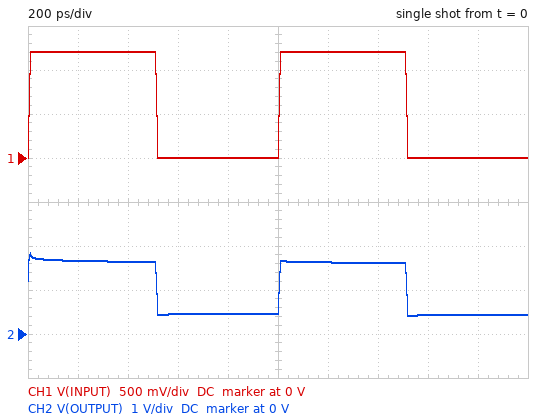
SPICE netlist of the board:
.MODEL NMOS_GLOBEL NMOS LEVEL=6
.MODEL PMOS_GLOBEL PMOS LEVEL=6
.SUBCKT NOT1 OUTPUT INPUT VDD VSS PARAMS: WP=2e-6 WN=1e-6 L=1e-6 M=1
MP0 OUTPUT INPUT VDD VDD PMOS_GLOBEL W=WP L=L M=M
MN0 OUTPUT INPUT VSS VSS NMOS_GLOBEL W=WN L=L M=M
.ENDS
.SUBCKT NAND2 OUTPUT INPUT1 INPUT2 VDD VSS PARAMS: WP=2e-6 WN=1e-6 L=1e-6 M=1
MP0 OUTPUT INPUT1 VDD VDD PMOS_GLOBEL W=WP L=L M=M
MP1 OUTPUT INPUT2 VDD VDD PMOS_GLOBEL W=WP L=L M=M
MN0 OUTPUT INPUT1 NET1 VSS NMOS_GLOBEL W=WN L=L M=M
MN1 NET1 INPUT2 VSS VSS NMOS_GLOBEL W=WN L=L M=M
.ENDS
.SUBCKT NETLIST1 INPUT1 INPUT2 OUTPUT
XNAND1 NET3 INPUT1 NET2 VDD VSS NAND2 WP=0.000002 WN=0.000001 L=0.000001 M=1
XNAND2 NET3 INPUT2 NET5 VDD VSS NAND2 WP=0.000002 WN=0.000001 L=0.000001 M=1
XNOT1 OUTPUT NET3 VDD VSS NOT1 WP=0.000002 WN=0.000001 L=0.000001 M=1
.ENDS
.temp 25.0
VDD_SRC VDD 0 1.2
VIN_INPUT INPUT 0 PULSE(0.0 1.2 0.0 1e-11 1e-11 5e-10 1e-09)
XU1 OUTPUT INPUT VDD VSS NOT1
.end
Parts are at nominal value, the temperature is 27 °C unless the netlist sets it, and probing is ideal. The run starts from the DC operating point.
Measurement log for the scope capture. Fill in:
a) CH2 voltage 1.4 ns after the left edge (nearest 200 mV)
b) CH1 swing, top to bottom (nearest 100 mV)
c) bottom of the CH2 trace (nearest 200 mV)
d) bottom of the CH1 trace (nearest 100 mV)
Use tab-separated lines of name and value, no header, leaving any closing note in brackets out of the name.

CH2 voltage 1.4 ns after the left edge	1.6 V
CH1 swing, top to bottom	1.2 V
bottom of the CH2 trace	400 mV
bottom of the CH1 trace	0 V
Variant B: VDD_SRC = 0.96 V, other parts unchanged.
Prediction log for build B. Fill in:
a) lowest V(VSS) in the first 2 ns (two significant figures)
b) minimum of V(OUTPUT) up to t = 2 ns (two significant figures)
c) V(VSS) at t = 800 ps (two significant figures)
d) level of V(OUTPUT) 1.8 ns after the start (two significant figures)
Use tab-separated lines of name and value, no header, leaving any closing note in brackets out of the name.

lowest V(VSS) in the first 2 ns	560 mV
minimum of V(OUTPUT) up to t = 2 ns	180 mV
V(VSS) at t = 800 ps	590 mV
level of V(OUTPUT) 1.8 ns after the start	190 mV
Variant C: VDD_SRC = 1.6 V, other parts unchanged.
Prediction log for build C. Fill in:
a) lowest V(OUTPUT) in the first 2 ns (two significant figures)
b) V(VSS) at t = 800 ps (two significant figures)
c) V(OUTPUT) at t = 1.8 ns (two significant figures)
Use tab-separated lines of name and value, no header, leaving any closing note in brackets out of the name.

lowest V(OUTPUT) in the first 2 ns	820 mV
V(VSS) at t = 800 ps	1.2 V
V(OUTPUT) at t = 1.8 ns	830 mV
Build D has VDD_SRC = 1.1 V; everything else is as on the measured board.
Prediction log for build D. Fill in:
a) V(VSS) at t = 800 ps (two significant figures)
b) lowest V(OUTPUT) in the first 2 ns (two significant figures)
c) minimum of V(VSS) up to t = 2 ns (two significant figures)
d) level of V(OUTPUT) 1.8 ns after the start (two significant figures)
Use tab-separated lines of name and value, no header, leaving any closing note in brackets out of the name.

V(VSS) at t = 800 ps	730 mV
lowest V(OUTPUT) in the first 2 ns	320 mV
minimum of V(VSS) up to t = 2 ns	700 mV
level of V(OUTPUT) 1.8 ns after the start	330 mV
